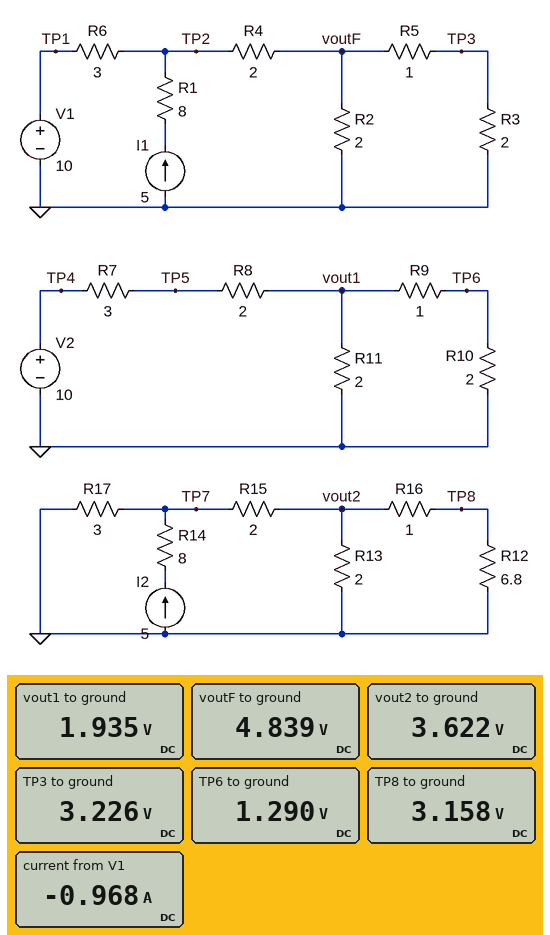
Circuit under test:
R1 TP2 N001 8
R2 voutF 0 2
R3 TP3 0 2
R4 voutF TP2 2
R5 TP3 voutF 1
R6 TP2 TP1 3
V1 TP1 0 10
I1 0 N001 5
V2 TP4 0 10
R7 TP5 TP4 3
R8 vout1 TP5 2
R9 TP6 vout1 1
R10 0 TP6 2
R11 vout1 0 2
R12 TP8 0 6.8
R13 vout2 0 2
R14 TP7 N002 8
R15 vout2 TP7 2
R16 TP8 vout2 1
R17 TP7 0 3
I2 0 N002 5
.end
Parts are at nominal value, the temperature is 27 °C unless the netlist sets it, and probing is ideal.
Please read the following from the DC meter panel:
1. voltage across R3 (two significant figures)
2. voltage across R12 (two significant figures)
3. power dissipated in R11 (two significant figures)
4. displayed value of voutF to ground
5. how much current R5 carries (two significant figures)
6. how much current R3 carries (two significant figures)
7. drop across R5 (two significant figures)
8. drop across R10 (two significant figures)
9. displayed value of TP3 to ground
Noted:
3.2 V
3.2 V
1.9 W
4.839 V
1.6 A
1.6 A
1.6 V
1.3 V
3.226 V
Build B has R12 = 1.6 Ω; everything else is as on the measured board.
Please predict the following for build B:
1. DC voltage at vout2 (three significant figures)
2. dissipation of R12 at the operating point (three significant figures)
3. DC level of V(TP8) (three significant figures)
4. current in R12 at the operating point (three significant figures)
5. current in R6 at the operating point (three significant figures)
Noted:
2.77 V
1.81 W
1.70 V
1.06 A
968 mA
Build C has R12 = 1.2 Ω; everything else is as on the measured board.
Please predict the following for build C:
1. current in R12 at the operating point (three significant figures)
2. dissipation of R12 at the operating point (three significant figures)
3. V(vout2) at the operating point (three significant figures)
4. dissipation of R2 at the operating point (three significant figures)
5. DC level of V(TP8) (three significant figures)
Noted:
1.18 A
1.67 W
2.60 V
11.7 W
1.42 V
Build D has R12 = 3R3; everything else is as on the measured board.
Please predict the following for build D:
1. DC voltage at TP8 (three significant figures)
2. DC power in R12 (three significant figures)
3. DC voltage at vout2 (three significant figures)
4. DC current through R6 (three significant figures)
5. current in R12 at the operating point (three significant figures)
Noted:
2.47 V
1.85 W
3.22 V
968 mA
748 mA
